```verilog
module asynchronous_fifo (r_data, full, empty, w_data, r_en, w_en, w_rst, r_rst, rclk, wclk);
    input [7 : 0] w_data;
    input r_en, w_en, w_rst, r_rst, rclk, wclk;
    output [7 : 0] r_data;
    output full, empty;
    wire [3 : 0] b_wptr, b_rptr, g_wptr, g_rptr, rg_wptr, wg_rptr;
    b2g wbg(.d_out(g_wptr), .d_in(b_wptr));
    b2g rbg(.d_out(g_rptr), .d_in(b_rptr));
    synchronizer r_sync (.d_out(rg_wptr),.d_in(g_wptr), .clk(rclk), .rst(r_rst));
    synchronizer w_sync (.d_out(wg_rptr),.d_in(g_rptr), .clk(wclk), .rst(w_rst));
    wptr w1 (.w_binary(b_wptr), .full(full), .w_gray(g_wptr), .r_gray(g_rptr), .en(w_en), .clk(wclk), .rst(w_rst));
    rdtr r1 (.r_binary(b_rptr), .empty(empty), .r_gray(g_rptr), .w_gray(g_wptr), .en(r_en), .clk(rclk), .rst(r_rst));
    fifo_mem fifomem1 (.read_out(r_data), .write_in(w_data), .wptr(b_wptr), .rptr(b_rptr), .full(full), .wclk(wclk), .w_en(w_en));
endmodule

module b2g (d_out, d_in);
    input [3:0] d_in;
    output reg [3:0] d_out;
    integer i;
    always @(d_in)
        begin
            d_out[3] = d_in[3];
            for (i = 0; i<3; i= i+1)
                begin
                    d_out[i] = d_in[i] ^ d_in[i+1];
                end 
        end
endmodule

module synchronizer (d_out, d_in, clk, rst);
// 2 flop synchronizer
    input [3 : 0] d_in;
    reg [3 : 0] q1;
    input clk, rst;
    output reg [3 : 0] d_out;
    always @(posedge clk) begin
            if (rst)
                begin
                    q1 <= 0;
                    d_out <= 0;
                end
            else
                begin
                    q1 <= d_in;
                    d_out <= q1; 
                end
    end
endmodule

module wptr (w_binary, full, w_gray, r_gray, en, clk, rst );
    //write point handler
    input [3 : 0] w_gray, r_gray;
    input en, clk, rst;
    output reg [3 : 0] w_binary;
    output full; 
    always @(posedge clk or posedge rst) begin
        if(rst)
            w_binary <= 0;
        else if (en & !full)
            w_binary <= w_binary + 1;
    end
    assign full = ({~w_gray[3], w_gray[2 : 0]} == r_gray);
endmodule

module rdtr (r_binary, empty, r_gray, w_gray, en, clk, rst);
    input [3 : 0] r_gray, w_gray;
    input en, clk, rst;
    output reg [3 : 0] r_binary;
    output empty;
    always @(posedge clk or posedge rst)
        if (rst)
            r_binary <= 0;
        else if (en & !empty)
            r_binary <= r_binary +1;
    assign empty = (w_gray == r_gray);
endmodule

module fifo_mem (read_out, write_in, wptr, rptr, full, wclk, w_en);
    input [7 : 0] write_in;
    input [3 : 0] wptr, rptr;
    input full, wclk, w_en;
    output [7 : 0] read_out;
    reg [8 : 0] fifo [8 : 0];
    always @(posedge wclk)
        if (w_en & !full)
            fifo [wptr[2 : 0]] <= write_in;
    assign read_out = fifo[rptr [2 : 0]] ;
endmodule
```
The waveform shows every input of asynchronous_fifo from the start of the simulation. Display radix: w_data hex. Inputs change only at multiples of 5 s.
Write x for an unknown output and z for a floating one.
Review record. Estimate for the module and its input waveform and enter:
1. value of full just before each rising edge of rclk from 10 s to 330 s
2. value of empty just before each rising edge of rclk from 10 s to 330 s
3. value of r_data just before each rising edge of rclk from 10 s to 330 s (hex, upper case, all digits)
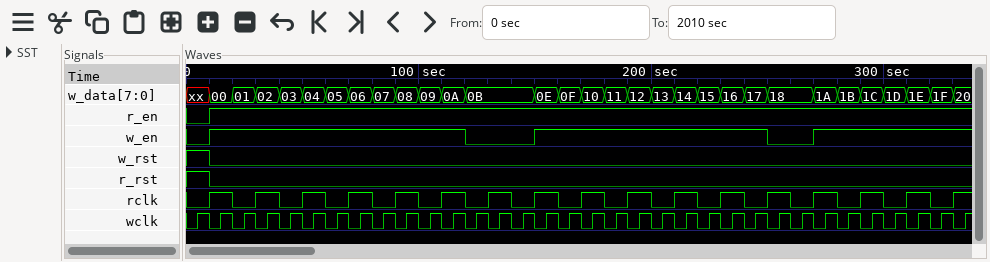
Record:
0 0 0 0 0 0 1 0 0 0 0 0 1 0 0 0 0
1 0 0 0 0 0 0 0 0 0 0 0 0 0 0 0 0
x, 00, 01, 02, 03, 04, 05, 06, 07, 08, 09, 0E, 17, 10, 1B, 1C, 1D
